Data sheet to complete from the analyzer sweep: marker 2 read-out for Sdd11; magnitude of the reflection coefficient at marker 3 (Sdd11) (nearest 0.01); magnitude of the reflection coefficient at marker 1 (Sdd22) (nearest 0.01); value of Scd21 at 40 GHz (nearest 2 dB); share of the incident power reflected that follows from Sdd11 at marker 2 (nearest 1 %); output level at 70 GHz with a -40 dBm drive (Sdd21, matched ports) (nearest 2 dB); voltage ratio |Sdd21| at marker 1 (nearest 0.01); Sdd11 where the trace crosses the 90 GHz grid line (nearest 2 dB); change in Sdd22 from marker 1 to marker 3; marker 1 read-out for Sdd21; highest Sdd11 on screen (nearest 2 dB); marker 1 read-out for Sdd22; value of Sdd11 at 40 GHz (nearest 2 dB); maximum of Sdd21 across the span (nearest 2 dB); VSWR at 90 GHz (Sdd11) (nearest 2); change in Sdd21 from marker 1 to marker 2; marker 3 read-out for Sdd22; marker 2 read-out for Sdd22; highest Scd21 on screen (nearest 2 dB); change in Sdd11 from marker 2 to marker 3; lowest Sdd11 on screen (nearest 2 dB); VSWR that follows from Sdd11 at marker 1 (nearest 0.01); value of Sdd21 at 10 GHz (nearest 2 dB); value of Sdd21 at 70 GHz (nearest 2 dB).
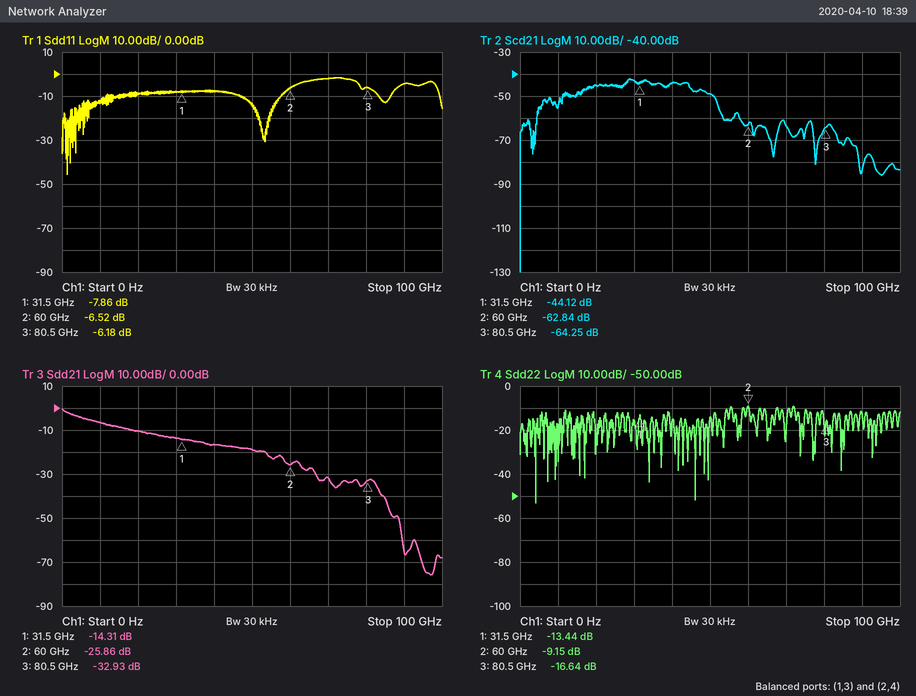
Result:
-6.52 dB
0.49
0.21
-44 dB
22 %
-72 dBm
0.19
-4 dB
-3.20 dB
-14.31 dB
-2 dB
-13.44 dB
-8 dB
0 dB
4
-11.55 dB
-16.64 dB
-9.15 dB
-42 dB
0.34 dB
-46 dB
2.36
-6 dB
-32 dB
